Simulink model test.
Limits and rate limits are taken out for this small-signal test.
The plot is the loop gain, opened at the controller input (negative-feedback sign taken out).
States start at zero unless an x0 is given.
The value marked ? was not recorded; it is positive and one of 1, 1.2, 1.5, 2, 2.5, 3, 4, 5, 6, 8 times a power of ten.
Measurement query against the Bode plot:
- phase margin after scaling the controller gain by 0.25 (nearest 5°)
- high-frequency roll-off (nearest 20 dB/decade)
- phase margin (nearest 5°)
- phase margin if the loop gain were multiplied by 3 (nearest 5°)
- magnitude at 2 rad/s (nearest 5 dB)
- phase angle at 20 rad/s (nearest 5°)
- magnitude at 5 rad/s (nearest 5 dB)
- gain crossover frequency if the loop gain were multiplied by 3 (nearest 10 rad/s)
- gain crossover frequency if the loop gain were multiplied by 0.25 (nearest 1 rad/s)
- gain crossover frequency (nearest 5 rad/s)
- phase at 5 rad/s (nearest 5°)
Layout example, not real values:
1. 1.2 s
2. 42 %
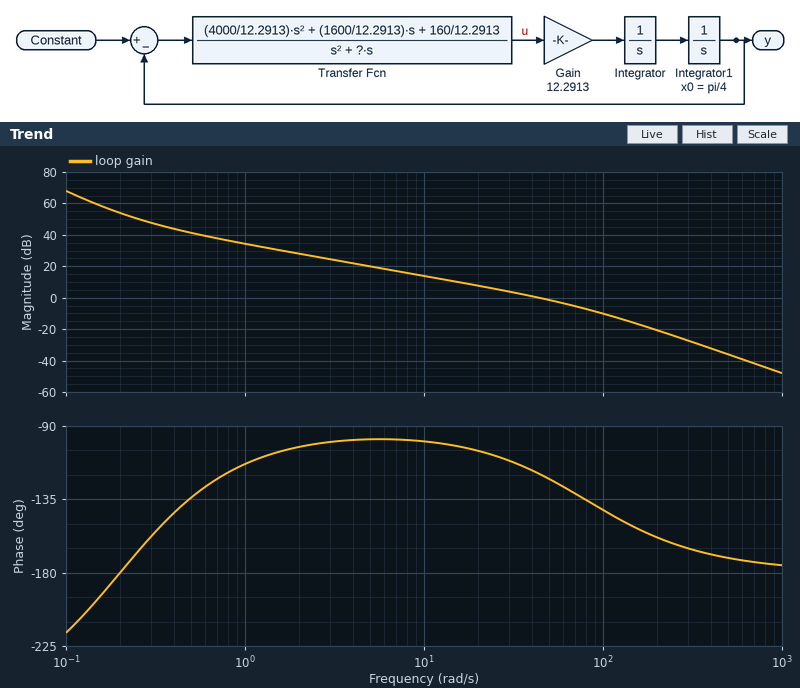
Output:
1. 80°
2. -40 dB/decade
3. 60°
4. 40°
5. 30 dB
6. -105°
7. 20 dB
8. 100 rad/s
9. 12 rad/s
10. 45 rad/s
11. -100°
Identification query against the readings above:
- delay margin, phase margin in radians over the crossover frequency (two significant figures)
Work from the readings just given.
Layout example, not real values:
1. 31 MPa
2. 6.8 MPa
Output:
1. 0.023 s
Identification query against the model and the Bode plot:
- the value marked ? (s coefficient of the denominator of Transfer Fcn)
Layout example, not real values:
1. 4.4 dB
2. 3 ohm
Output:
1. 80
